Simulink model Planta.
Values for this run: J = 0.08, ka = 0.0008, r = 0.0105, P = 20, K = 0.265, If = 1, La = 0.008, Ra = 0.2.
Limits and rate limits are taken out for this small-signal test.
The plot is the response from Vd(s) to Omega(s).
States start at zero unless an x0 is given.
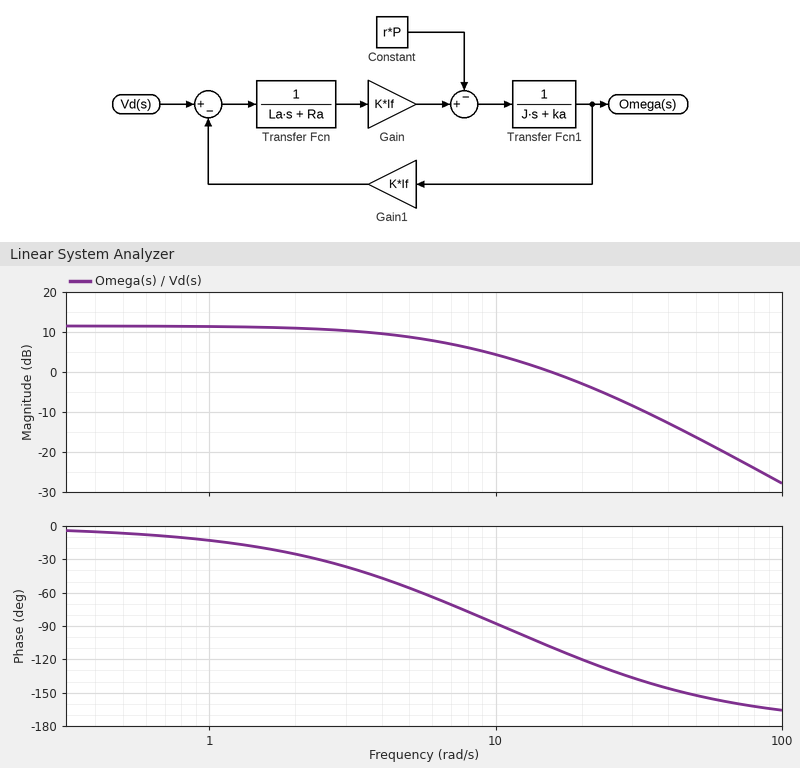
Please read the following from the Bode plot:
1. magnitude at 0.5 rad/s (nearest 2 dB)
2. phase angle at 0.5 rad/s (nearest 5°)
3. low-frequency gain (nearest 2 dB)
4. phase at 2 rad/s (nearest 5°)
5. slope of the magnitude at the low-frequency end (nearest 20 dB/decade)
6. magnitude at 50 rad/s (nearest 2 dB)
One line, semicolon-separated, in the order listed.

12 dB; -5°; 12 dB; -25°; 0 dB/decade; -16 dB
